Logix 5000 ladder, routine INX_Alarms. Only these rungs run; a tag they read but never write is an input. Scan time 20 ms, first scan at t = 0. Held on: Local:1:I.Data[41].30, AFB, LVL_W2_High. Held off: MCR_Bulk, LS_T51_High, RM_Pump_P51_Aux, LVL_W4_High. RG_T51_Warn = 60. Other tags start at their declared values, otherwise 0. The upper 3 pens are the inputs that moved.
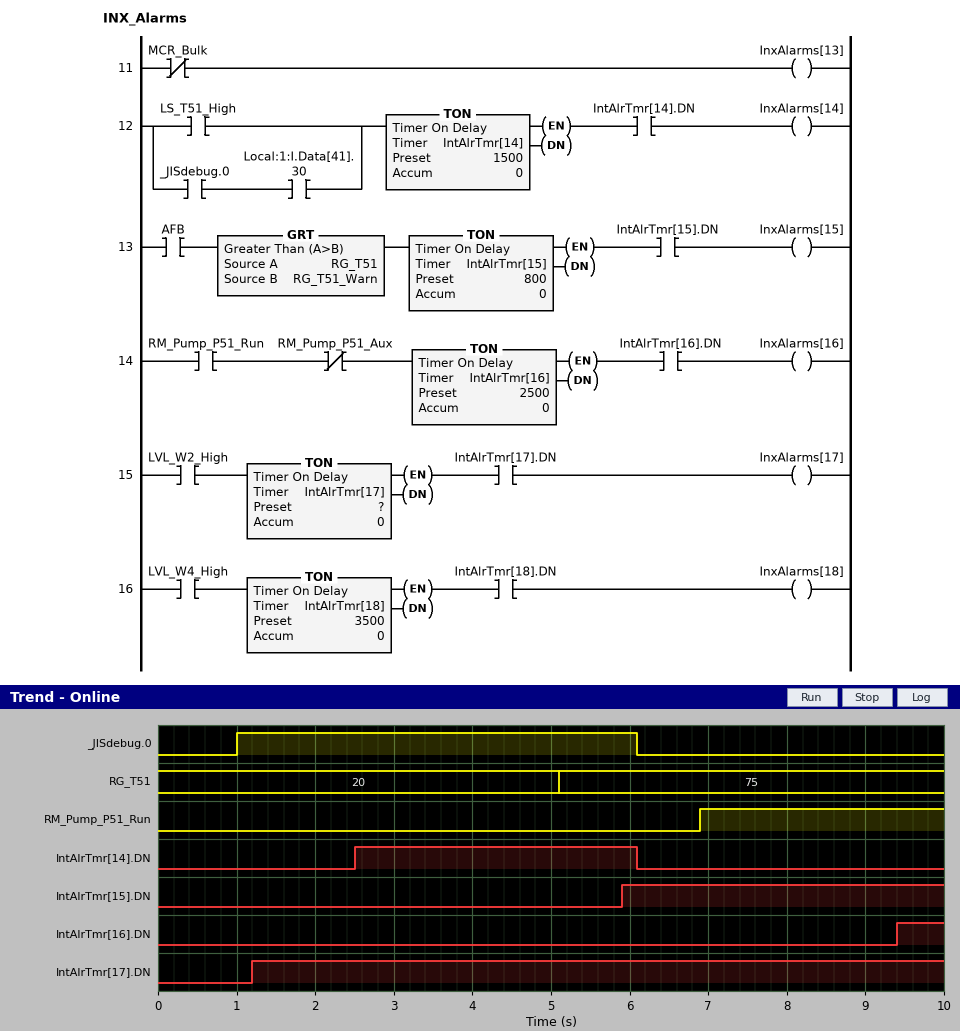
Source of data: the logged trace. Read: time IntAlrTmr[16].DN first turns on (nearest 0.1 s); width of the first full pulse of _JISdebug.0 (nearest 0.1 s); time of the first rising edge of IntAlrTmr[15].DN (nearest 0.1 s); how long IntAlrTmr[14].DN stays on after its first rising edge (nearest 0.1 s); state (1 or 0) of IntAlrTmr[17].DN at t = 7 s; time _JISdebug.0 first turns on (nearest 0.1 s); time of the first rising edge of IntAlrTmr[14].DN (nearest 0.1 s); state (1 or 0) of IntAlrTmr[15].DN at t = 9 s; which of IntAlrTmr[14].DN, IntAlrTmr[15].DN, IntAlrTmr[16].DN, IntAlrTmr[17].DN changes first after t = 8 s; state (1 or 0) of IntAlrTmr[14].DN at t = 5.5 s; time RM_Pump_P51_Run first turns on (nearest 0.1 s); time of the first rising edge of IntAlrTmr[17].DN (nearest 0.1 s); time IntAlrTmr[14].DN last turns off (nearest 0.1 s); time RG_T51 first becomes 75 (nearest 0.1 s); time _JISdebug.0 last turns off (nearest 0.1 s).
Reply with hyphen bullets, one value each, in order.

- 9.4 s
- 5.1 s
- 5.9 s
- 3.6 s
- 1
- 1.0 s
- 2.5 s
- 1
- IntAlrTmr[16].DN
- 1
- 6.9 s
- 1.2 s
- 6.1 s
- 5.1 s
- 6.1 s
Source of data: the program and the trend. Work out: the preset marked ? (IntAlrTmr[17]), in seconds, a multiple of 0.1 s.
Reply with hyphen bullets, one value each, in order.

- 1.2 s
